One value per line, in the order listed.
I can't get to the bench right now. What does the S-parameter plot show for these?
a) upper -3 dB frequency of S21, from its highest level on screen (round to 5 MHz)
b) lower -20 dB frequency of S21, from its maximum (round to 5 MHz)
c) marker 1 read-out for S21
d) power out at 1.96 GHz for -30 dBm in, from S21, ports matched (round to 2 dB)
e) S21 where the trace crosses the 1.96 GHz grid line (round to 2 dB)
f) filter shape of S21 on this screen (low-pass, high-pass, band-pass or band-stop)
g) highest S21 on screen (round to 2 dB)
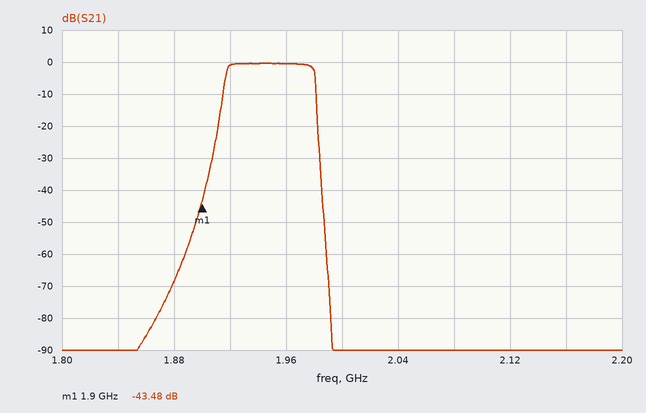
1.980 GHz
1.910 GHz
-43.48 dB
-30 dBm
0 dB
band-pass
0 dB
